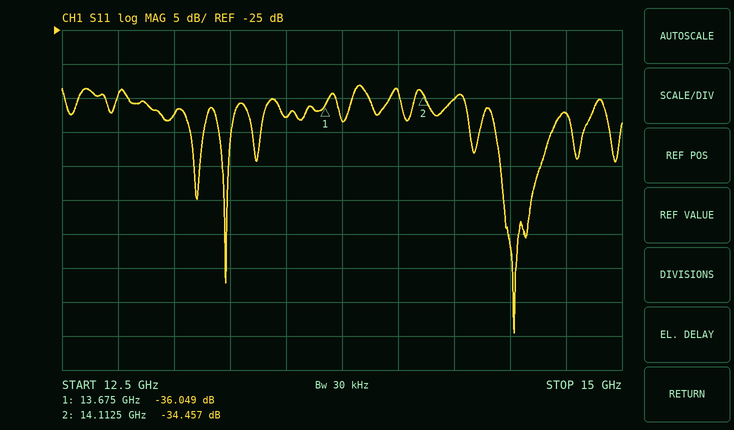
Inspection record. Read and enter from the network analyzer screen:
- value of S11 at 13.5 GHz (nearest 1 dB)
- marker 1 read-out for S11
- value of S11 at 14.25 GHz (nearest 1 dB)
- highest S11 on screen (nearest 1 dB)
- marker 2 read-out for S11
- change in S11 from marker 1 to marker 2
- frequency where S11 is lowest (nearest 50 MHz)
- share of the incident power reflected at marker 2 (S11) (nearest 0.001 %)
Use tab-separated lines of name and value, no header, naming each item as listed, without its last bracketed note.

value of S11 at 13.5 GHz	-38 dB
marker 1 read-out for S11	-36.049 dB
value of S11 at 14.25 GHz	-35 dB
highest S11 on screen	-33 dB
marker 2 read-out for S11	-34.457 dB
change in S11 from marker 1 to marker 2	1.592 dB
frequency where S11 is lowest	14.50 GHz
share of the incident power reflected at marker 2 (S11)	0.036 %
